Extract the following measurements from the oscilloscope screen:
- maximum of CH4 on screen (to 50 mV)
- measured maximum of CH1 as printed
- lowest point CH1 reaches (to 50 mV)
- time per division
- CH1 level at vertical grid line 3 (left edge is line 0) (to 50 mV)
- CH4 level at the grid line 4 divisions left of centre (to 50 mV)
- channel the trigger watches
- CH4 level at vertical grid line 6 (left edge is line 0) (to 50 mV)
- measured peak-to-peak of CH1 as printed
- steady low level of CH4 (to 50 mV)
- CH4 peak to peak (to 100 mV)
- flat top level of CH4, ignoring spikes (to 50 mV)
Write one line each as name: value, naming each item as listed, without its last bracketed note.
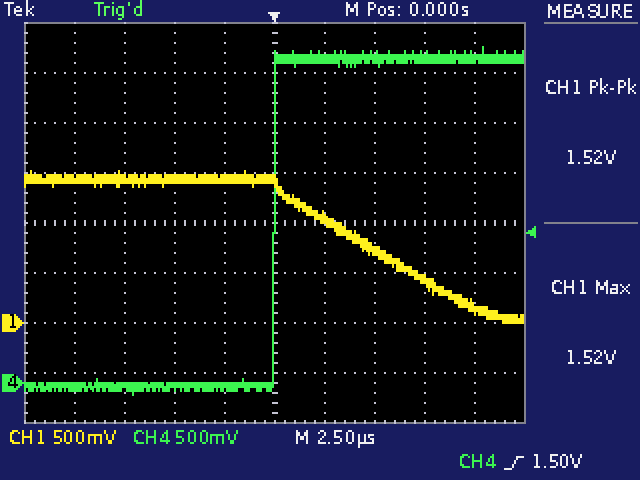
maximum of CH4 on screen: 3.35 V
measured maximum of CH1 as printed: 1.52 V
lowest point CH1 reaches: 0 mV
time per division: 2.5 µs
CH1 level at vertical grid line 3 (left edge is line 0): 1.45 V
CH4 level at the grid line 4 divisions left of centre: -50 mV
channel the trigger watches: CH4
CH4 level at vertical grid line 6 (left edge is line 0): 3.25 V
measured peak-to-peak of CH1 as printed: 1.52 V
steady low level of CH4: -50 mV
CH4 peak to peak: 3.50 V
flat top level of CH4, ignoring spikes: 3.25 V
